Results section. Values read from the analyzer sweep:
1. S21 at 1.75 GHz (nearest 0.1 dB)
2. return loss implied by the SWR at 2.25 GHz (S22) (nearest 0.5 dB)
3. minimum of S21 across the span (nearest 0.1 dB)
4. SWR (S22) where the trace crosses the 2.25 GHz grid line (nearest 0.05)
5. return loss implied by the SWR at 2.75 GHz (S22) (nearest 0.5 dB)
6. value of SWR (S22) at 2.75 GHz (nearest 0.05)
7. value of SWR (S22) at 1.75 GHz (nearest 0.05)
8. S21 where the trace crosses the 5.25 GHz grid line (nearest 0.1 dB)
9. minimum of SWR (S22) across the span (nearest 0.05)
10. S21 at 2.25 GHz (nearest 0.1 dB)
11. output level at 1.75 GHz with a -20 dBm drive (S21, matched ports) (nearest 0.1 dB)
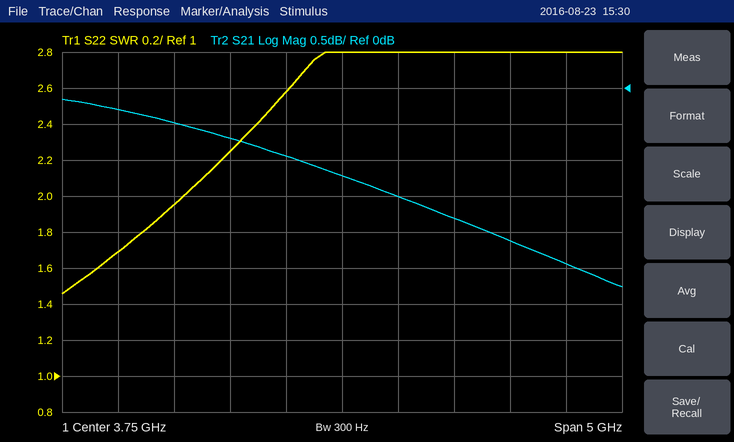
-0.3 dB
10.0 dB
-2.8 dB
1.95
8.5 dB
2.25
1.70
-2.1 dB
1.45
-0.5 dB
-20.3 dBm
